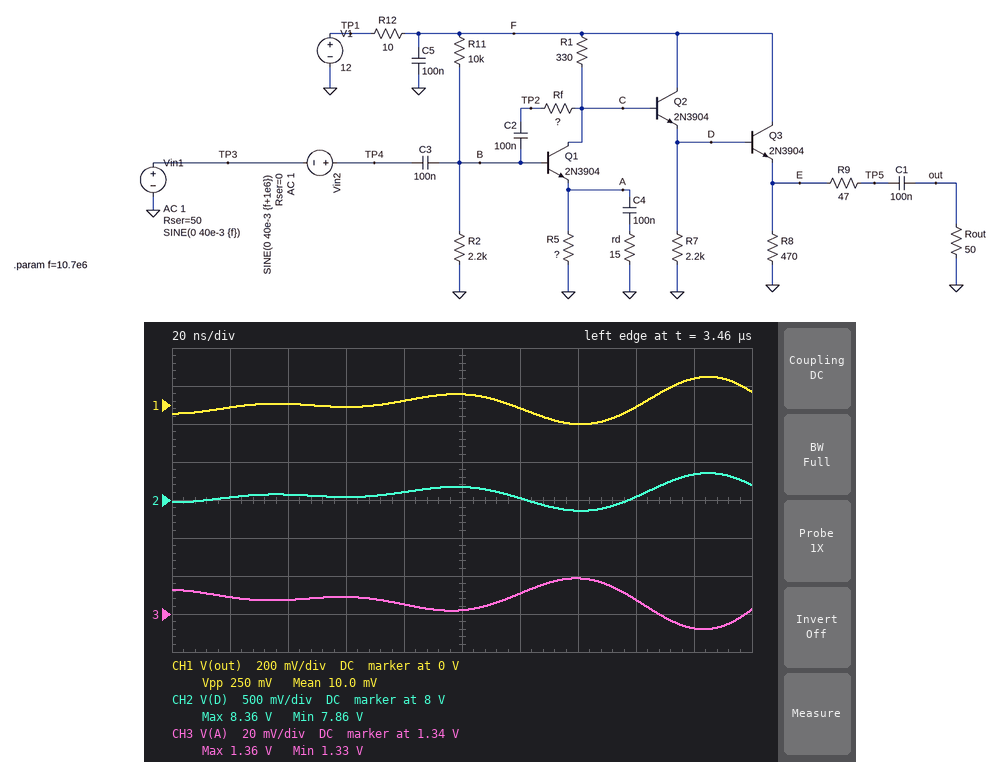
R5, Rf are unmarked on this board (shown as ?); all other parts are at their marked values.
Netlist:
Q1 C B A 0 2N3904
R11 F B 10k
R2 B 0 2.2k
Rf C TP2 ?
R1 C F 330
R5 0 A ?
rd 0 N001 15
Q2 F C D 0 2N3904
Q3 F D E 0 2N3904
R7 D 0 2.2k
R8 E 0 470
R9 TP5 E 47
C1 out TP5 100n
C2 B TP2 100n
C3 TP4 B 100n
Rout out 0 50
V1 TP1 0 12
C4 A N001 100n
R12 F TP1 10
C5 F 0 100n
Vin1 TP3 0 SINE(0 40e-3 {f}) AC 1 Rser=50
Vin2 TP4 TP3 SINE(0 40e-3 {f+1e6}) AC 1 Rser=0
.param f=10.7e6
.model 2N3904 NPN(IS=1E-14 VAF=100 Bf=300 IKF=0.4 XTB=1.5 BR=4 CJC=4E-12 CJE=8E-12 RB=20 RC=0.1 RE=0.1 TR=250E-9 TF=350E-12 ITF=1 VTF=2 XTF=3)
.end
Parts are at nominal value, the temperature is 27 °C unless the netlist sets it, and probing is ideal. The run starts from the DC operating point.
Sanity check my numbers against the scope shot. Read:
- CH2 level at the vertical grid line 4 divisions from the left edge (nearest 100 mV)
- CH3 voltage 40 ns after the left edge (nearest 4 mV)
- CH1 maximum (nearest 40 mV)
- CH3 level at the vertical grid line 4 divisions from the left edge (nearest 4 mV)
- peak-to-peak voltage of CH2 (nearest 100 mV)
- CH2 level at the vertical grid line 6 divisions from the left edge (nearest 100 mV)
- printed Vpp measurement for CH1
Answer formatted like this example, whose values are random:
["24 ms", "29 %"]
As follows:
["8.1 V", "1.348 V", "160 mV", "1.344 V", "500 mV", "8.0 V", "250 mV"]
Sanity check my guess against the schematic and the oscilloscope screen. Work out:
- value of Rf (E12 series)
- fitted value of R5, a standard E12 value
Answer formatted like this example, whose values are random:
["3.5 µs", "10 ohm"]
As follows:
["1.2 kΩ", "150 Ω"]
